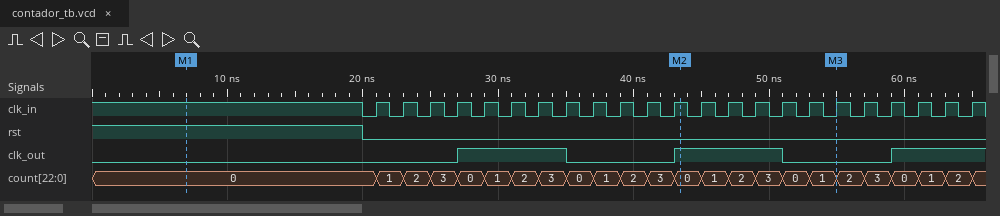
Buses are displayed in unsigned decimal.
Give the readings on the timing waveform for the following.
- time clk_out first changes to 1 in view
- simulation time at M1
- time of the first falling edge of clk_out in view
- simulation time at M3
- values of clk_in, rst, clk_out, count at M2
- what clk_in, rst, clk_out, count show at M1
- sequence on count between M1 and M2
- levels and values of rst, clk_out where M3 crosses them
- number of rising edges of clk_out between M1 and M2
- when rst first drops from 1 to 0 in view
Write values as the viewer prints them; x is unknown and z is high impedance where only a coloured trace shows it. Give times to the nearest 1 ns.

27 ns
7 ns
35 ns
55 ns
clk_in=1, rst=0, clk_out=1, count=0
clk_in=1, rst=1, clk_out=0, count=0
0, 1, 2, 3, 0, 1, 2, 3, 0, 1, 2, 3, 0
rst=0, clk_out=0
2
20 ns
